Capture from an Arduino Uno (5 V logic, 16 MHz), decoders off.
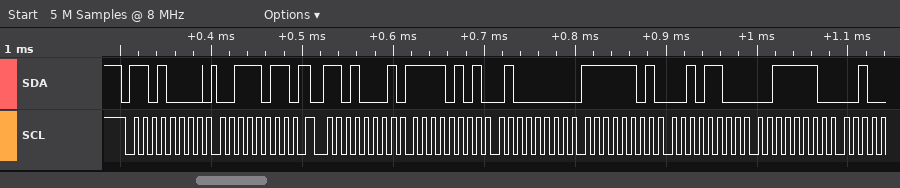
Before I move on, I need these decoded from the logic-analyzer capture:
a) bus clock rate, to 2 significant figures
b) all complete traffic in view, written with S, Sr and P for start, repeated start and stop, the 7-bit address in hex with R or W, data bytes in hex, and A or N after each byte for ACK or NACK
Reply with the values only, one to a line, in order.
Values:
100 kHz
S 68W A 3B A Sr 68R A F5 A 40 A FD A 2C A 3E A
